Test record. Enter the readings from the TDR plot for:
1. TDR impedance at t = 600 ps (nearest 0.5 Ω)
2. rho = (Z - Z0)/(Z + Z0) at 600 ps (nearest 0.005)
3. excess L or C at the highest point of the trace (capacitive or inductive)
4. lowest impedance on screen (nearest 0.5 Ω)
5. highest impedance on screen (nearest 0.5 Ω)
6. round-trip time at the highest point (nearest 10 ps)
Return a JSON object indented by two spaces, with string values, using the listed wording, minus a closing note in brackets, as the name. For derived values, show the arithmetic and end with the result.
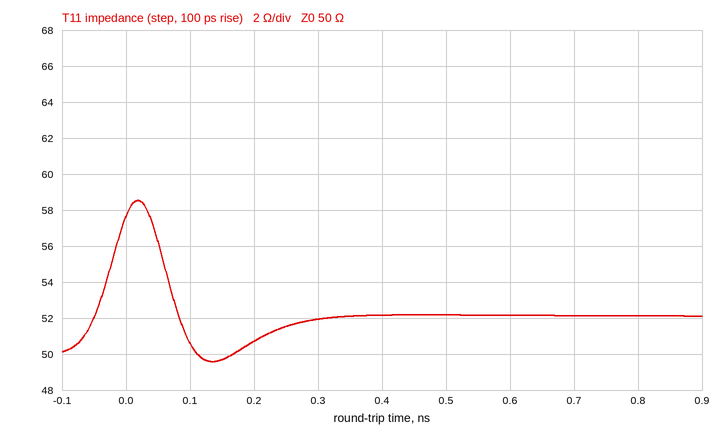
{
  "TDR impedance at t = 600 ps": "52.0 Ω",
  "rho = (Z - Z0)/(Z + Z0) at 600 ps": "(52 − 50)/(52 + 50) ≈ +0.020",
  "excess L or C at the highest point of the trace": "inductive",
  "lowest impedance on screen": "49.5 Ω",
  "highest impedance on screen": "58.5 Ω",
  "round-trip time at the highest point": "20 ps"
}
